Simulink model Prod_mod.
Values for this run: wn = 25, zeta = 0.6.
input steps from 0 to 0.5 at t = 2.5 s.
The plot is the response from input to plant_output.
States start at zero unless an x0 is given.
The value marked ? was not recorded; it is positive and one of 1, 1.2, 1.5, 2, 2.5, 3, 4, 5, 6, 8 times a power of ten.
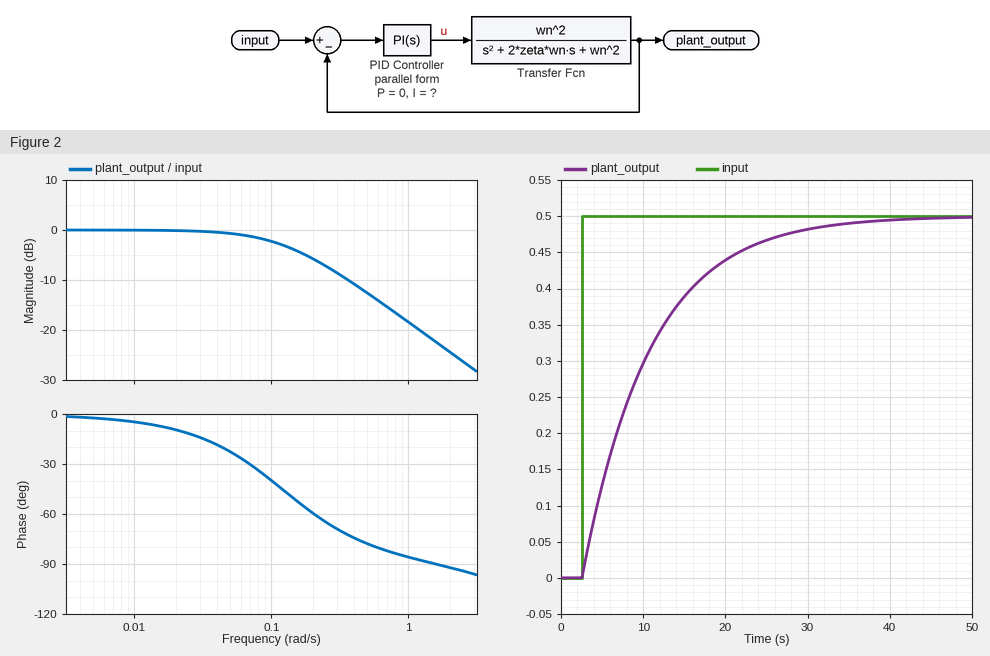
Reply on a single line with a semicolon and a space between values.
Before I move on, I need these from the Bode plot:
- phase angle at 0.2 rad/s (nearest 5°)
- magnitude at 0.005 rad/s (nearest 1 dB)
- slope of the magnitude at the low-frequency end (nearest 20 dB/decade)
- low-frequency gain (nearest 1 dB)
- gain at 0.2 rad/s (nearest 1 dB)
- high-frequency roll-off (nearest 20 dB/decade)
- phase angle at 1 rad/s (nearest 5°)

-60°; 0 dB; 0 dB/decade; 0 dB; -6 dB; -20 dB/decade; -85°
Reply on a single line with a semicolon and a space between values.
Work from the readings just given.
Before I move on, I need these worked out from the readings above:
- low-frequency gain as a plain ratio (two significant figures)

1.0
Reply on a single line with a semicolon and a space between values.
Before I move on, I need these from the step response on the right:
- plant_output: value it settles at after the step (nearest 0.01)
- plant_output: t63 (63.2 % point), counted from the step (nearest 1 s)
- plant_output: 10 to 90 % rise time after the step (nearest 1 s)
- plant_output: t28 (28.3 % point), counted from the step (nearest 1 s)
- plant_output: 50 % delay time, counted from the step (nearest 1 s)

0.50; 8 s; 18 s; 3 s; 6 s
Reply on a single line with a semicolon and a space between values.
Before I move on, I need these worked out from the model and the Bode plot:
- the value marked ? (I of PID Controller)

0.12
